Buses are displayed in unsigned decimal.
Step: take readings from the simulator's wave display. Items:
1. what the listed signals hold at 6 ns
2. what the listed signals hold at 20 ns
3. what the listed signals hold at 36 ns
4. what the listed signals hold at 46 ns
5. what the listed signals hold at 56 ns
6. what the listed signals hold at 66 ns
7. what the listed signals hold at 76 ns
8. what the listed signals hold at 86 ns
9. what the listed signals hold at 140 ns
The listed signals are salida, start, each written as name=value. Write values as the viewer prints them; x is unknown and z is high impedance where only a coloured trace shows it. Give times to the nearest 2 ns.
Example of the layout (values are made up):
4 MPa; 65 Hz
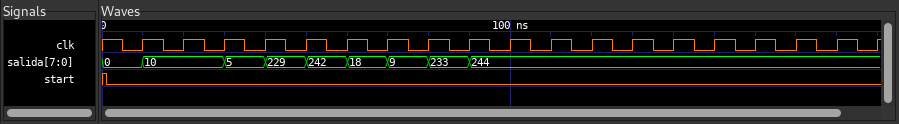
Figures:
salida=0, start=0; salida=10, start=0; salida=5, start=0; salida=229, start=0; salida=242, start=0; salida=18, start=0; salida=9, start=0; salida=233, start=0; salida=244, start=0
